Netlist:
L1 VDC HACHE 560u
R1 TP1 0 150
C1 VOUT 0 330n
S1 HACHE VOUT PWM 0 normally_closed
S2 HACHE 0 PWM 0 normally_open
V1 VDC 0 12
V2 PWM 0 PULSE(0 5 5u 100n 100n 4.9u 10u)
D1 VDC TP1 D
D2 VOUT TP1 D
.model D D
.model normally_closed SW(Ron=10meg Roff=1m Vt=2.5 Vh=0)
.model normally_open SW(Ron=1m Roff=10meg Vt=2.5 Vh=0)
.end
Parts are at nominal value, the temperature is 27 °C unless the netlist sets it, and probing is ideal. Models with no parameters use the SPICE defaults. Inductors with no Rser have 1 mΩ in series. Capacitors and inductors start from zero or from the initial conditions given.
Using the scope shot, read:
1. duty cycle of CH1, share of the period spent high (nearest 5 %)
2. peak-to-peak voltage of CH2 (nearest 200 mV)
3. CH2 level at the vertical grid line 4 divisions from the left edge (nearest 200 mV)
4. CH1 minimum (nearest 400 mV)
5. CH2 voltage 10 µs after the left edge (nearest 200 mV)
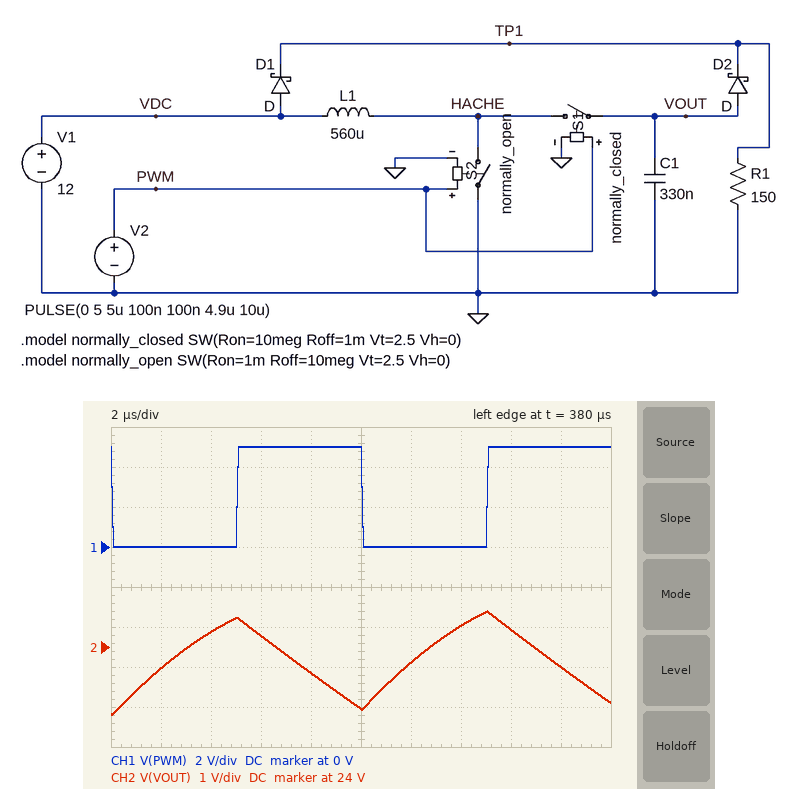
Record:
50 %
2.6 V
23.4 V
0 V
22.4 V
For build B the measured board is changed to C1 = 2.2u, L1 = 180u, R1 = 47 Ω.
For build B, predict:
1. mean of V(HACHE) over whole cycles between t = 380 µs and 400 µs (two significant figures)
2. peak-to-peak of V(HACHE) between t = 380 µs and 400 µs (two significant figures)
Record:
14 V
28 V
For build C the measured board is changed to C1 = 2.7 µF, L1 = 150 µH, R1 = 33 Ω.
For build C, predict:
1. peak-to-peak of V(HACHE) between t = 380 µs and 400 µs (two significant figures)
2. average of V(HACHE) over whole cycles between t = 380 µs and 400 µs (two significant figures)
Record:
27 V
13 V
